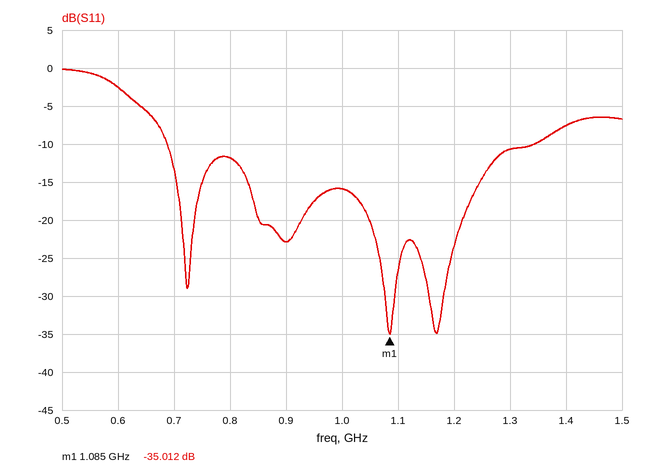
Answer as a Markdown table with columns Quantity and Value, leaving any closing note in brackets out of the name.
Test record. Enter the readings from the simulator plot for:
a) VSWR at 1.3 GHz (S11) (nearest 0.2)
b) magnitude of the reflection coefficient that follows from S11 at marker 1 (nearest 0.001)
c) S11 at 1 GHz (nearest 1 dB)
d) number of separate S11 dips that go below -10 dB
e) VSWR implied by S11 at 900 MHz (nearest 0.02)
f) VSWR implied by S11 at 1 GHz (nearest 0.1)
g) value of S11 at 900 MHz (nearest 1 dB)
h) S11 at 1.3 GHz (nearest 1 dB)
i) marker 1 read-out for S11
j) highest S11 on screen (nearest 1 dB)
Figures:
| Quantity | Value |
|---|---|
| VSWR at 1.3 GHz (S11) | 1.8 |
| magnitude of the reflection coefficient that follows from S11 at marker 1 | 0.018 |
| S11 at 1 GHz | -16 dB |
| number of separate S11 dips that go below -10 dB | 4 |
| VSWR implied by S11 at 900 MHz | 1.16 |
| VSWR implied by S11 at 1 GHz | 1.4 |
| value of S11 at 900 MHz | -23 dB |
| S11 at 1.3 GHz | -11 dB |
| marker 1 read-out for S11 | -35.012 dB |
| highest S11 on screen | 0 dB |
